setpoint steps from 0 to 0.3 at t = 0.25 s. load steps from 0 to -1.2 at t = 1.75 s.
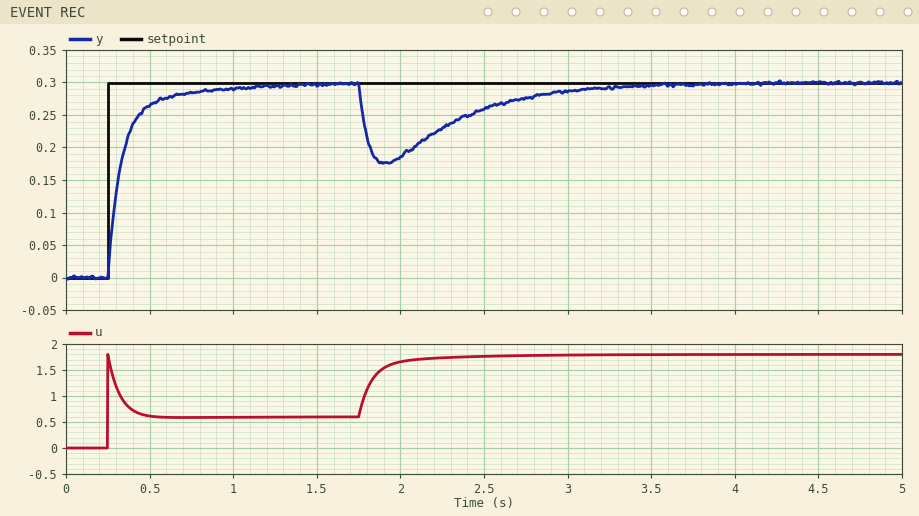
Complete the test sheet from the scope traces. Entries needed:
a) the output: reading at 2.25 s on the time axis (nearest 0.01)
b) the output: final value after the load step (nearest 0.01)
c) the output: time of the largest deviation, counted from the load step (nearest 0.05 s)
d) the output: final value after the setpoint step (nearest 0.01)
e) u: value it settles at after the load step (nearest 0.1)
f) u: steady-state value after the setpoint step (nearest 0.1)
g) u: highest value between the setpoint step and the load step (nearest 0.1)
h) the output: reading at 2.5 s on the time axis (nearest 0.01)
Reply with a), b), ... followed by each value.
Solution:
a) 0.23
b) 0.30
c) 0.15 s
d) 0.30
e) 1.8
f) 0.6
g) 1.8
h) 0.26
